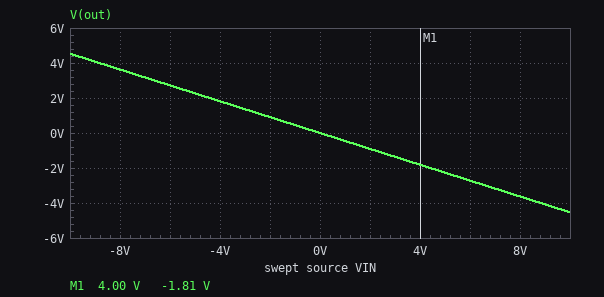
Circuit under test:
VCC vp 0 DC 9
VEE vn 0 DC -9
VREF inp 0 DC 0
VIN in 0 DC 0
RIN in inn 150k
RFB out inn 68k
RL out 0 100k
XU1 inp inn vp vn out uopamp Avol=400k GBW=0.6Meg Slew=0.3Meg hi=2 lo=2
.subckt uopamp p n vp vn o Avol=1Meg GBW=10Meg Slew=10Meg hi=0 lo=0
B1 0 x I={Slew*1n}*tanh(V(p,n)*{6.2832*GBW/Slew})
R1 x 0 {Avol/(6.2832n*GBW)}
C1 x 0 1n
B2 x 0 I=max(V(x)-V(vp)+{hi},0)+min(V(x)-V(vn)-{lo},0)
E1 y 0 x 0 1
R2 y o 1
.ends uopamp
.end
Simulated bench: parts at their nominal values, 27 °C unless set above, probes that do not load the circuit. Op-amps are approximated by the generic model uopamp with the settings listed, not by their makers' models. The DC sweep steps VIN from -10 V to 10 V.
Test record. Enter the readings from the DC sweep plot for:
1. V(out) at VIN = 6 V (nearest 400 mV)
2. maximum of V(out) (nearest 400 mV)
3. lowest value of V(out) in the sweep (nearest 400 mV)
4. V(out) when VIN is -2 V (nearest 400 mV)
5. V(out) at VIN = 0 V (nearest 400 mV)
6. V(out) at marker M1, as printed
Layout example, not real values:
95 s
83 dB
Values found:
-2.8 V
4.4 V
-4.4 V
800 mV
0 V
-1.81 V
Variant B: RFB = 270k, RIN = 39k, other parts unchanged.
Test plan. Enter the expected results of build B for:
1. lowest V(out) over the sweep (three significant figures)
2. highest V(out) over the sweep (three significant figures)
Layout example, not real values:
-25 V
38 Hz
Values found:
-7.00 V
7.00 V
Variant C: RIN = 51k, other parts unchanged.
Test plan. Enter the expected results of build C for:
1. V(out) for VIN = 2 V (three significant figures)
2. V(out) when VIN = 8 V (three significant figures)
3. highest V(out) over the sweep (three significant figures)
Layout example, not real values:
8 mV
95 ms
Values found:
-2.67 V
-7.00 V
7.00 V
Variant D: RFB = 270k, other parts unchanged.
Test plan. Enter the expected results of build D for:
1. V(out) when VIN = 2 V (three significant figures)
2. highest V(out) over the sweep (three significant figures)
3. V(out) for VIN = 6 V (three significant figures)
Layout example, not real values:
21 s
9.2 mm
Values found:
-3.60 V
7.00 V
-7.00 V
